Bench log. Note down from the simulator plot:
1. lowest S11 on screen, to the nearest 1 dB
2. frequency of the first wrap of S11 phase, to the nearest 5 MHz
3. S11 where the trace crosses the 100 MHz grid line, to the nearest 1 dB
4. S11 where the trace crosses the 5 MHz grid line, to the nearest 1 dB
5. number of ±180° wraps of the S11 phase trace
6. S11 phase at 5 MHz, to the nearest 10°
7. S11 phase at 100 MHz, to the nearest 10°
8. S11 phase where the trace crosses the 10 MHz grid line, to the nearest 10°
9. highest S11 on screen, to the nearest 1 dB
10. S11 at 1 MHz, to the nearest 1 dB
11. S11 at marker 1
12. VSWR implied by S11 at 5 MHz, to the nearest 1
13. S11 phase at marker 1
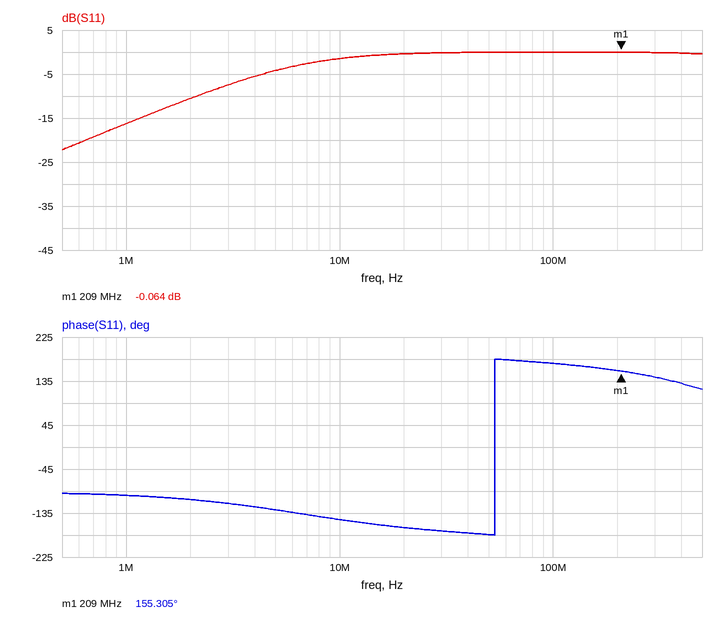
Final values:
-22 dB
55 MHz
0 dB
-4 dB
1
-130°
170°
-150°
0 dB
-16 dB
-0.064 dB
4
155.305°
